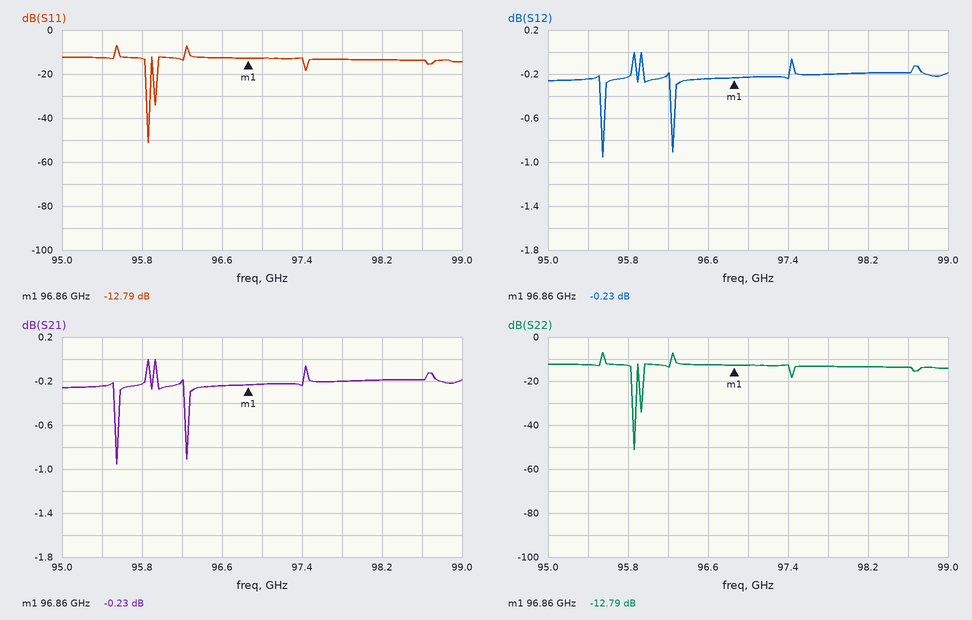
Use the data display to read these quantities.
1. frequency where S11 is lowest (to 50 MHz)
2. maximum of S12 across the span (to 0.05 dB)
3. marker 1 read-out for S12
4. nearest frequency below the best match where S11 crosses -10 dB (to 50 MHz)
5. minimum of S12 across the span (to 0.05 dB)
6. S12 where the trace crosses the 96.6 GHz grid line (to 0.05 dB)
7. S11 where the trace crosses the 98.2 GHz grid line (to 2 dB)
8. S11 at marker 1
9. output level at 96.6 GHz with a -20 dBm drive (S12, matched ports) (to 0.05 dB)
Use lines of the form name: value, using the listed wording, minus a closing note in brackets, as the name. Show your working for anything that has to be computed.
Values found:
frequency where S11 is lowest: 95.85 GHz
maximum of S12 across the span: 0.00 dB
marker 1 read-out for S12: -0.23 dB
nearest frequency below the best match where S11 crosses -10 dB: 95.55 GHz
minimum of S12 across the span: -0.95 dB
S12 where the trace crosses the 96.6 GHz grid line: -0.25 dB
S11 where the trace crosses the 98.2 GHz grid line: -14 dB
S11 at marker 1: -12.79 dB
output level at 96.6 GHz with a -20 dBm drive (S12, matched ports): -20 dBm + (-0.25 dB) = -20.25 dBm
